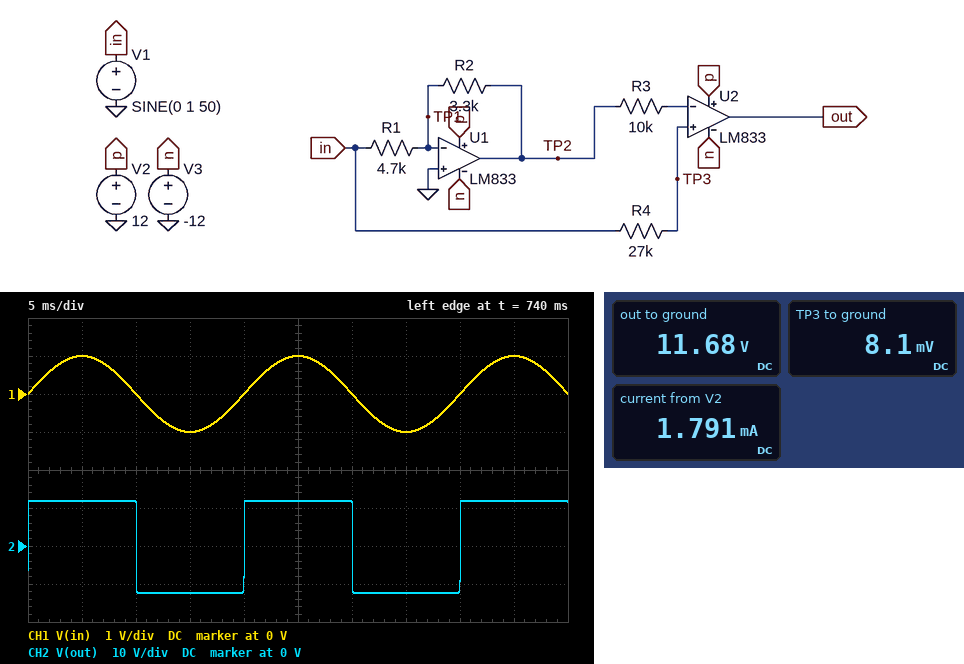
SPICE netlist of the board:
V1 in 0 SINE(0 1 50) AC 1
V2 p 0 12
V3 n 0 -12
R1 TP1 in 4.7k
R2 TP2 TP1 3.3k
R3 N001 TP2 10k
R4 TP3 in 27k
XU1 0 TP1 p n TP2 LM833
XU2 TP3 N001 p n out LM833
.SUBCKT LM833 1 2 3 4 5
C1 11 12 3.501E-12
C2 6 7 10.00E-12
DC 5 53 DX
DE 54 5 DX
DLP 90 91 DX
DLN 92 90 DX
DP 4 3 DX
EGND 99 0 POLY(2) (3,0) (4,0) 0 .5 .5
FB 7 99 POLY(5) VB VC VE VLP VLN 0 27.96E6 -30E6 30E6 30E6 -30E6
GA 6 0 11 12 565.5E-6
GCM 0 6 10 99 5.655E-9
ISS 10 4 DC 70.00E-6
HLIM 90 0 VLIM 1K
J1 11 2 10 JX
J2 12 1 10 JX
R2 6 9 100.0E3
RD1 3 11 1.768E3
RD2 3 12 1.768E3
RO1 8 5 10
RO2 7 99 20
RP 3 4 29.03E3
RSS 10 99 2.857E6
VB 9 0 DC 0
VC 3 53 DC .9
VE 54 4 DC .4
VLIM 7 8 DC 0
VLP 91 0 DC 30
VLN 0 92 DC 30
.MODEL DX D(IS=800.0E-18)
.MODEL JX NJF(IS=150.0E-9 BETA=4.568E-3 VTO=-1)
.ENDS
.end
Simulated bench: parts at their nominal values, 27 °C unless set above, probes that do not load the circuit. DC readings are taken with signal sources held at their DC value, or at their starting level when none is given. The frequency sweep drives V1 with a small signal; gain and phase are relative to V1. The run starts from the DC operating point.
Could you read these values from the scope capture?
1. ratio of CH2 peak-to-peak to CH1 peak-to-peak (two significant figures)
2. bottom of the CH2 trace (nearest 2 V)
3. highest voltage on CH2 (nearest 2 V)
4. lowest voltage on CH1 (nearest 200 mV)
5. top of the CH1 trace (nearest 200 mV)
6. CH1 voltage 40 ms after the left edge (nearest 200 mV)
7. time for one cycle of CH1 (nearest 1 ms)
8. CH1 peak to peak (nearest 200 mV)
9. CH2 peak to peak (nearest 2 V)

12
-12 V
12 V
-1.0 V
1.0 V
0 V
20 ms
2.0 V
24 V
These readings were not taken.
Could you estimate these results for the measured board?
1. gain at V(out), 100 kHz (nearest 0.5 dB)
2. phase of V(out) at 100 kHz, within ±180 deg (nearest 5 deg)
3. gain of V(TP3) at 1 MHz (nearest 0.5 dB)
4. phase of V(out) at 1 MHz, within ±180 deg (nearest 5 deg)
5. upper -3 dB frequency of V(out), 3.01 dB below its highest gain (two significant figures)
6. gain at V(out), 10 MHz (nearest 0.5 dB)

15.5 dB
-35 deg
0 dB
-90 deg
150 kHz
-25.0 dB
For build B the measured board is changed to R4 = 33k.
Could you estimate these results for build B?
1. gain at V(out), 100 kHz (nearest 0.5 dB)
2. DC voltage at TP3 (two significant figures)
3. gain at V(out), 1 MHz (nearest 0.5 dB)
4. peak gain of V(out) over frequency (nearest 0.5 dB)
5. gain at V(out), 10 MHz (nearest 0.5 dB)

13.5 dB
9.9 mV
-1.5 dB
15.0 dB
-27.0 dB
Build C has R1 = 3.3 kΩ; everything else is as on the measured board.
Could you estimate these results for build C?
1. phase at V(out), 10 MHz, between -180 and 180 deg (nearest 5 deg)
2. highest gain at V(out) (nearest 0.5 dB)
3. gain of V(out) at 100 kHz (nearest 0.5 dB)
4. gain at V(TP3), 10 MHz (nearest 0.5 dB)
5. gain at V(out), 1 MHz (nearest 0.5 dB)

-160 deg
18.5 dB
17.0 dB
0 dB
2.0 dB
